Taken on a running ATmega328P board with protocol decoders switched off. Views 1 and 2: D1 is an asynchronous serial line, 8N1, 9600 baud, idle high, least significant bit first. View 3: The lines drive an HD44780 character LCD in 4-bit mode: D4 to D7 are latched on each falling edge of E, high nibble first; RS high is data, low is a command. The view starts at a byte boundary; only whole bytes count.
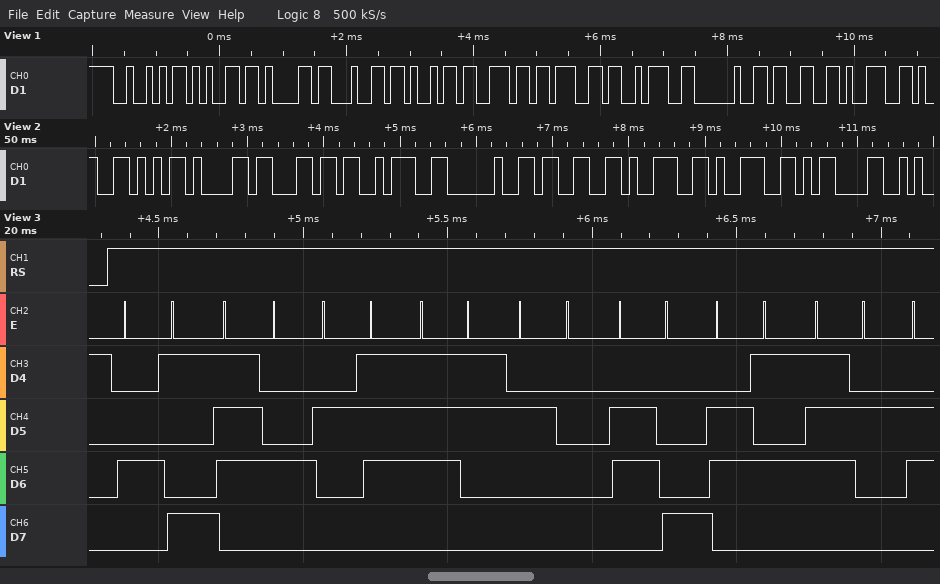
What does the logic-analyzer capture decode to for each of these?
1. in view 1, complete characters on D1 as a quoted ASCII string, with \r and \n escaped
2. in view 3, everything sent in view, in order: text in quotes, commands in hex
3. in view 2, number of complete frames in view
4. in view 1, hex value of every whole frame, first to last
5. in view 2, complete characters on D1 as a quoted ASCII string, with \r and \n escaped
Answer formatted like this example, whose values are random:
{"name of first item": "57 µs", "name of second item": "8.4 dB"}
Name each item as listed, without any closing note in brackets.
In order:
{"in view 1, complete characters on D1 as a quoted ASCII string, with \\r and \\n escaped": "\"Reading: 39\"", "in view 3, everything sent in view, in order: text in quotes, commands in hex": "\"It's her\"", "in view 2, number of complete frames in view": "9", "in view 1, hex value of every whole frame, first to last": "52 65 61 64 69 6E 67 3A 20 33 39", "in view 2, complete characters on D1 as a quoted ASCII string, with \\r and \\n escaped": "\"Val: 399\\r\""}
